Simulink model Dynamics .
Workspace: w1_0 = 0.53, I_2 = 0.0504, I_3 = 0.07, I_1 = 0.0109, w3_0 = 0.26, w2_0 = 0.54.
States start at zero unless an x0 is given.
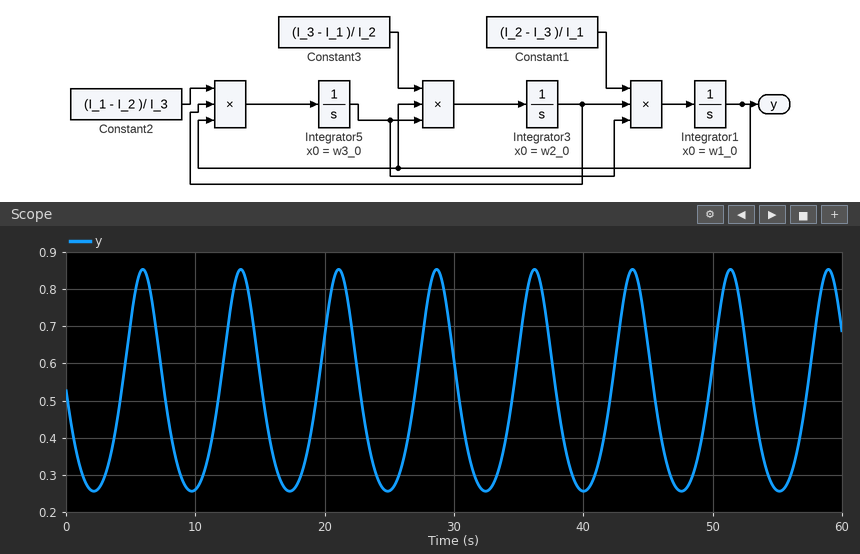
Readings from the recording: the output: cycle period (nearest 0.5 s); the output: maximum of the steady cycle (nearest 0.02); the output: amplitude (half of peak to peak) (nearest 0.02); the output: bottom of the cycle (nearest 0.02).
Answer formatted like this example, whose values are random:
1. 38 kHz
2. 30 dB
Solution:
1. 7.5 s
2. 0.86
3. 0.30
4. 0.26
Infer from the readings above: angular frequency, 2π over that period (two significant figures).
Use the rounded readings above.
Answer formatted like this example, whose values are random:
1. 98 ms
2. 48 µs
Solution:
1. 0.84 rad/s
